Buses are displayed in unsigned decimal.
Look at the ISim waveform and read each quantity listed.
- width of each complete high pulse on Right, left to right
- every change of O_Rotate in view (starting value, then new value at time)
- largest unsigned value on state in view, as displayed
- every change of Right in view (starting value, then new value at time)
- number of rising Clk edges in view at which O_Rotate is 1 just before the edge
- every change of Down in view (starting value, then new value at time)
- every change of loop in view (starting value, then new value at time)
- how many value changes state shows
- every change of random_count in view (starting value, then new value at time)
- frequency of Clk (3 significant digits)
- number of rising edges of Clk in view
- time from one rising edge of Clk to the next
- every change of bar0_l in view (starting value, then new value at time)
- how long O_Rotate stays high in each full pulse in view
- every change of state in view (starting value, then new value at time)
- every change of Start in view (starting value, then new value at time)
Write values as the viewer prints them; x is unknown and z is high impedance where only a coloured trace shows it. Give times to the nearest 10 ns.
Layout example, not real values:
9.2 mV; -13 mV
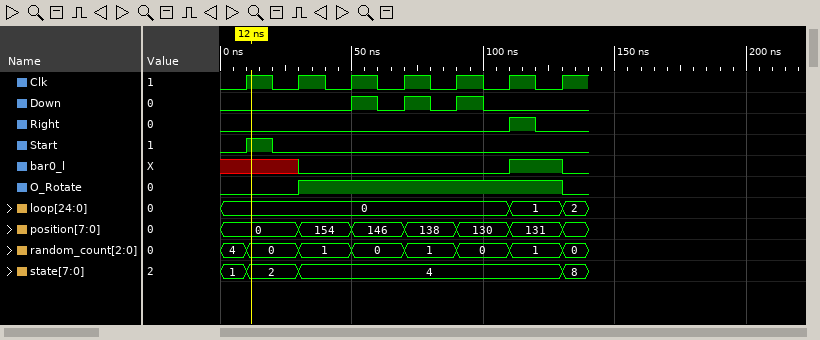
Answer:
10 ns; 0, 1 at 30 ns, 0 at 130 ns; 8; 0, 1 at 110 ns, 0 at 120 ns; 5; 0, 1 at 50 ns, 0 at 60 ns, 1 at 70 ns, 0 at 80 ns, 1 at 90 ns, 0 at 100 ns; 0, 1 at 110 ns, 2 at 130 ns; 3; 4, 0 at 10 ns, 1 at 30 ns, 0 at 50 ns, 1 at 70 ns, 0 at 90 ns, 1 at 110 ns, 0 at 130 ns; 50.0 MHz; 7; 20 ns; x, 0 at 30 ns, 1 at 110 ns, 0 at 130 ns; 100 ns; 1, 2 at 10 ns, 4 at 30 ns, 8 at 130 ns; 0, 1 at 10 ns, 0 at 20 ns
